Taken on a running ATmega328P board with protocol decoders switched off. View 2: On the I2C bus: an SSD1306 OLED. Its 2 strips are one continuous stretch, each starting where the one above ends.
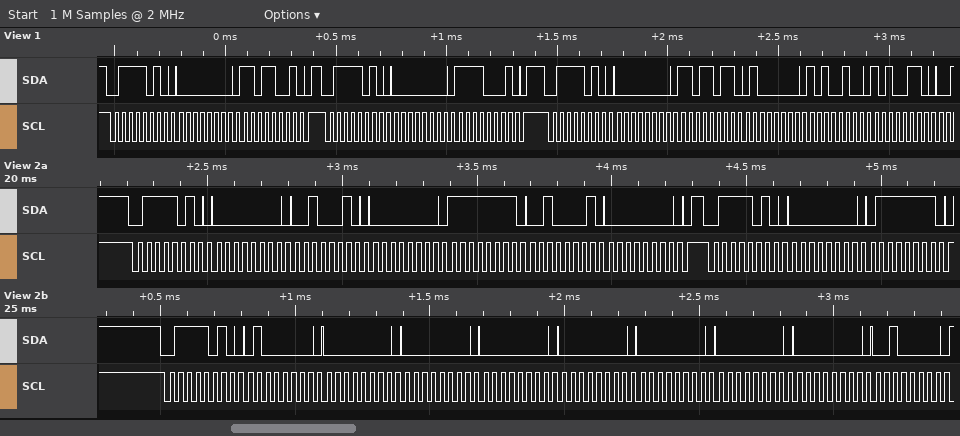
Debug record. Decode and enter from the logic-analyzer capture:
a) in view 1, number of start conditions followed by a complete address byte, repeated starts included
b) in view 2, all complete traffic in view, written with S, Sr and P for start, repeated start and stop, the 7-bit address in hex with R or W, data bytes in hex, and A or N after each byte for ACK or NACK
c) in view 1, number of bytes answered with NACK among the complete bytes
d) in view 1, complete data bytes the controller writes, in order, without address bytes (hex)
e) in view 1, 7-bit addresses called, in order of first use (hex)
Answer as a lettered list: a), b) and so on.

a) 3
b) S 3DW A 00 A 22 A 00 A FF A 21 A 00 A P S 3DW A 00 A 7F A P S 3DW A 40 A 00 A 00 A 00 A 00 A 00 A 00 A 00 A 20 A
c) 0
d) 00 D9 00 F1 00 DB 40 A4 A6
e) 0x3D
